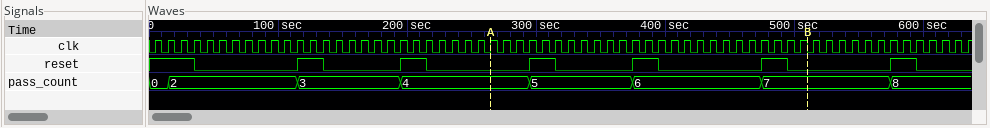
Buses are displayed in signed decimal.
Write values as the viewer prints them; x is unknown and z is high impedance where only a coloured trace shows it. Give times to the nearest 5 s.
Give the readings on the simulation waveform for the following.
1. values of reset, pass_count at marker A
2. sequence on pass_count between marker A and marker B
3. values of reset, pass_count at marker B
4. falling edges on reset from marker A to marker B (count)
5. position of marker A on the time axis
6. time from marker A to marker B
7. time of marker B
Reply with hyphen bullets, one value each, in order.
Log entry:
- reset=0, pass_count=4
- 4, 5, 6, 7
- reset=0, pass_count=7
- 3
- 265 s
- 245 s
- 510 s
